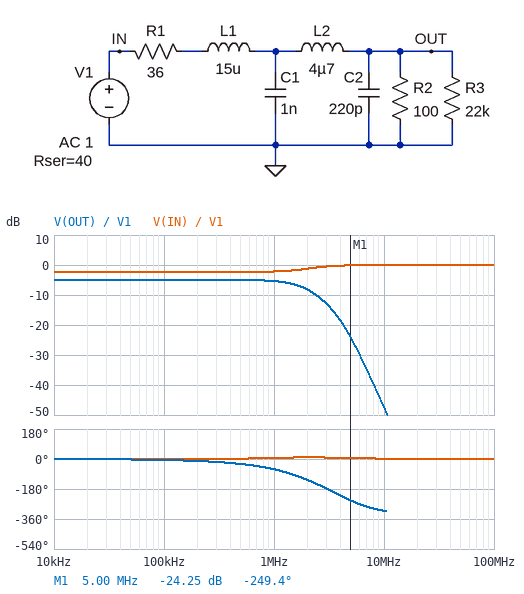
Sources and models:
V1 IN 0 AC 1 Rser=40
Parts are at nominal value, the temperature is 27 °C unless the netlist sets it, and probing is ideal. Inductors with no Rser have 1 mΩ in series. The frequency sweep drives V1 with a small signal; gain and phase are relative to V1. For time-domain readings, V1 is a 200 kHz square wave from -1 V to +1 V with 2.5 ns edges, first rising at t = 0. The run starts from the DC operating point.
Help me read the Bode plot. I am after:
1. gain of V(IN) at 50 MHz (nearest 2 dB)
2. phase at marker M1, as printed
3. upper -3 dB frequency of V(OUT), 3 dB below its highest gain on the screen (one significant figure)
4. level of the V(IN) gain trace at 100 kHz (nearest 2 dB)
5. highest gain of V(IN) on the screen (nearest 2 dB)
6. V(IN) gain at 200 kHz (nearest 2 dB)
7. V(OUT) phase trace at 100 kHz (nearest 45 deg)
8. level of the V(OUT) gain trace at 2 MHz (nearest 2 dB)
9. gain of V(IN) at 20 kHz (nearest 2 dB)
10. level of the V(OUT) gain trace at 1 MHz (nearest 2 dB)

0 dB
-249.4 deg
2 MHz
-2 dB
0 dB
-2 dB
0 deg
-8 dB
-2 dB
-6 dB
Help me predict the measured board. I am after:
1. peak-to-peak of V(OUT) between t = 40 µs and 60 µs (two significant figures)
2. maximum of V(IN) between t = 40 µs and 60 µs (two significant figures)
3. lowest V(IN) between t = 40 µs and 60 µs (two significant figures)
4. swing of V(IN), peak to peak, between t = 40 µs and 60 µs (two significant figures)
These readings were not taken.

1.2 V
1.2 V
-1.2 V
2.4 V
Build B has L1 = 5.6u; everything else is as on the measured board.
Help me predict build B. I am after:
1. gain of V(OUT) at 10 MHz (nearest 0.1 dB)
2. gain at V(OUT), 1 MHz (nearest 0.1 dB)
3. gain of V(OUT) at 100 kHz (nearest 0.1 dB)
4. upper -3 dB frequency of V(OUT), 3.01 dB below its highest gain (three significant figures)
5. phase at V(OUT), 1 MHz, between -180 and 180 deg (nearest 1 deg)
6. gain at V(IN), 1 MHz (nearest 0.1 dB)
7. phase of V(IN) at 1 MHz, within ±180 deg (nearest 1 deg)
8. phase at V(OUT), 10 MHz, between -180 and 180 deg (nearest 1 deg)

-38.7 dB
-4.9 dB
-4.9 dB
3.46 MHz
-41 deg
-2.5 dB
0 deg
57 deg
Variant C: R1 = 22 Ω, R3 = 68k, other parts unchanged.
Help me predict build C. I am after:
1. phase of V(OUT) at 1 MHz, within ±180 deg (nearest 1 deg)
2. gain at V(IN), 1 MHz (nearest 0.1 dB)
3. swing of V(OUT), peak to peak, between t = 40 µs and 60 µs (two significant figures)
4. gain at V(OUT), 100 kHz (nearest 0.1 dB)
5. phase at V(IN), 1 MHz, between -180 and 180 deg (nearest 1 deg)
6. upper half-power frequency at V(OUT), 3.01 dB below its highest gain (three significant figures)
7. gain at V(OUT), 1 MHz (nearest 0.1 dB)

-63 deg
-2.3 dB
1.3 V
-4.2 dB
7 deg
1.89 MHz
-4.6 dB
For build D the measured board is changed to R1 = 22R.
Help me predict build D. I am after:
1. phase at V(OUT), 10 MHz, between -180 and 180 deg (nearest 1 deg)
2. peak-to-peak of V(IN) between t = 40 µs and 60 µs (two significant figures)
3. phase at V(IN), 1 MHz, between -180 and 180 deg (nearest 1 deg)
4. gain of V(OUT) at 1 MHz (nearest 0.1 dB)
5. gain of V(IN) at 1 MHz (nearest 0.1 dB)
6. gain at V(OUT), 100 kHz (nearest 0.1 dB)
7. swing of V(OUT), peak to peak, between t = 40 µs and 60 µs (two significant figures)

48 deg
2.5 V
7 deg
-4.7 dB
-2.3 dB
-4.2 dB
1.3 V
